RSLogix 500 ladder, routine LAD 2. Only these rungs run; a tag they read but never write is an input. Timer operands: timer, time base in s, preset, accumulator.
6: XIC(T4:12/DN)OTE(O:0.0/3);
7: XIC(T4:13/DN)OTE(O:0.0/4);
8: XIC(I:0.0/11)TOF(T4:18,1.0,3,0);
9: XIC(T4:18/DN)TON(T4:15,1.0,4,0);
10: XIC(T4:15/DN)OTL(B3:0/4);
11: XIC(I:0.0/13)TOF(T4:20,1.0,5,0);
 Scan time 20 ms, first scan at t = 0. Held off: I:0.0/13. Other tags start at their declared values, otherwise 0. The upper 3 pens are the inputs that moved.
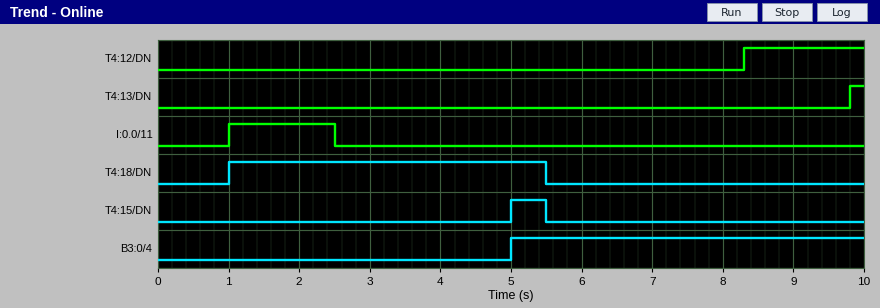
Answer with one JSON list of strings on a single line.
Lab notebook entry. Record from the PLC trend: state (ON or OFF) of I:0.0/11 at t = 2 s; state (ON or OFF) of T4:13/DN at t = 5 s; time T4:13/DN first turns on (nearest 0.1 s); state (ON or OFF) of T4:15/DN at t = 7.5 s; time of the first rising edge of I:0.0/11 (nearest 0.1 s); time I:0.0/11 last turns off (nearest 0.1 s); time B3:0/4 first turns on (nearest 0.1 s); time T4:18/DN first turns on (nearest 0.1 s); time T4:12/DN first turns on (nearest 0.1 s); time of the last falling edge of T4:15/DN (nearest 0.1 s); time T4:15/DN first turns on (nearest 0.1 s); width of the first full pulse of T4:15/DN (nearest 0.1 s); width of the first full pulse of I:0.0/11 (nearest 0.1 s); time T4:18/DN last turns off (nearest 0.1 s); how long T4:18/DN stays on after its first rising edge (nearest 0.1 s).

["ON", "OFF", "9.8 s", "OFF", "1.0 s", "2.5 s", "5.0 s", "1.0 s", "8.3 s", "5.5 s", "5.0 s", "0.5 s", "1.5 s", "5.5 s", "4.5 s"]
